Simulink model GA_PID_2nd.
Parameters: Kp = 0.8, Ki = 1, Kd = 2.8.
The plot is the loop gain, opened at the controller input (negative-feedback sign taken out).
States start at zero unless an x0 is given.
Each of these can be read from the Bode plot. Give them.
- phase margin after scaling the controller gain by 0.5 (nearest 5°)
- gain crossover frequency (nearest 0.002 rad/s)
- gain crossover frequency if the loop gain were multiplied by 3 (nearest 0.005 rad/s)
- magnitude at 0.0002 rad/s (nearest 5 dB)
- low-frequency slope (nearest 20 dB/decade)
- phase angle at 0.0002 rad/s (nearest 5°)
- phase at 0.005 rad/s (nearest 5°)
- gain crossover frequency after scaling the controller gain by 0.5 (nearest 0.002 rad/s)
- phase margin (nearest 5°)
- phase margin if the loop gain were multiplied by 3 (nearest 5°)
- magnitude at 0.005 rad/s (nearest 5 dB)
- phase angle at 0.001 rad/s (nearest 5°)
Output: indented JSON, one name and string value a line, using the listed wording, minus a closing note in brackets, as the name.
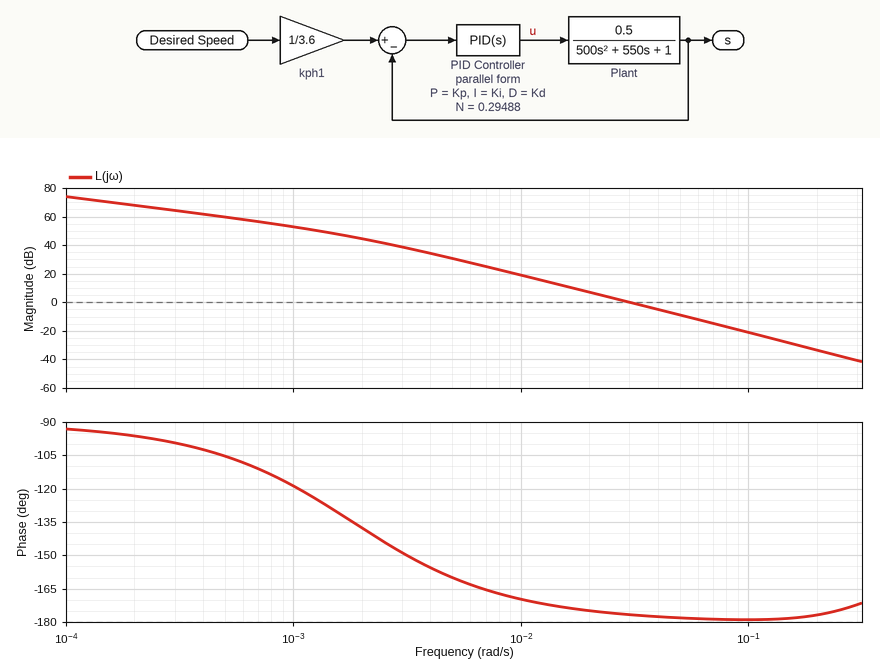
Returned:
{
  "phase margin after scaling the controller gain by 0.5": "5°",
  "gain crossover frequency": "0.030 rad/s",
  "gain crossover frequency if the loop gain were multiplied by 3": "0.050 rad/s",
  "magnitude at 0.0002 rad/s": "70 dB",
  "low-frequency slope": "-20 dB/decade",
  "phase angle at 0.0002 rad/s": "-95°",
  "phase at 0.005 rad/s": "-160°",
  "gain crossover frequency after scaling the controller gain by 0.5": "0.022 rad/s",
  "phase margin": "5°",
  "phase margin if the loop gain were multiplied by 3": "0°",
  "magnitude at 0.005 rad/s": "30 dB",
  "phase angle at 0.001 rad/s": "-120°"
}
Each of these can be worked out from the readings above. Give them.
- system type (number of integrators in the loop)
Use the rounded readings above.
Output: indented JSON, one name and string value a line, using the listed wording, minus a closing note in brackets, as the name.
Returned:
{
  "system type": "1"
}
